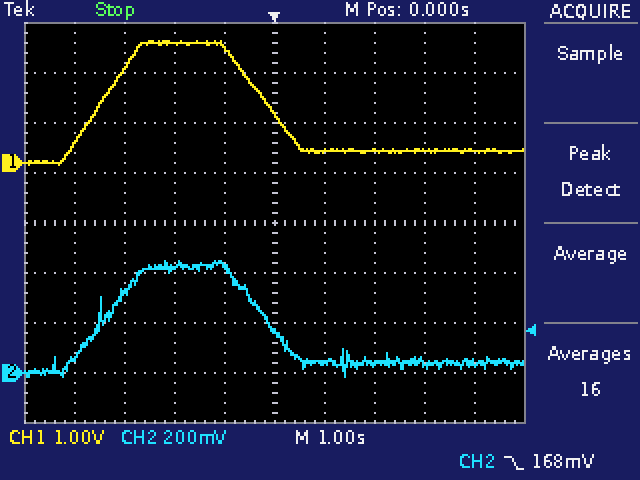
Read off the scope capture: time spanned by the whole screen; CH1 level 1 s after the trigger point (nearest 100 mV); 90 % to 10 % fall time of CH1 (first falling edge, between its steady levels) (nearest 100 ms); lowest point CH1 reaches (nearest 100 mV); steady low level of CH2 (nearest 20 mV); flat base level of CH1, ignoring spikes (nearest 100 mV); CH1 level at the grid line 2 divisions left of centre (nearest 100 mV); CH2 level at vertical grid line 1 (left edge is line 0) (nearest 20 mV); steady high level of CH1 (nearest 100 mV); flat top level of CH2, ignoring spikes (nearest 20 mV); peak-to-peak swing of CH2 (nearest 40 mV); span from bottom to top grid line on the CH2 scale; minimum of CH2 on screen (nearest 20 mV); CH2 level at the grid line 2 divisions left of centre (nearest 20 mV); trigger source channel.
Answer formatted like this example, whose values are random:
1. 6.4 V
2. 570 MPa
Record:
1. 10 s
2. 200 mV
3. 1.3 s
4. 0.0 V
5. 40 mV
6. 200 mV
7. 2.4 V
8. 60 mV
9. 2.4 V
10. 420 mV
11. 480 mV
12. 1.6 V
13. -20 mV
14. 420 mV
15. CH2
